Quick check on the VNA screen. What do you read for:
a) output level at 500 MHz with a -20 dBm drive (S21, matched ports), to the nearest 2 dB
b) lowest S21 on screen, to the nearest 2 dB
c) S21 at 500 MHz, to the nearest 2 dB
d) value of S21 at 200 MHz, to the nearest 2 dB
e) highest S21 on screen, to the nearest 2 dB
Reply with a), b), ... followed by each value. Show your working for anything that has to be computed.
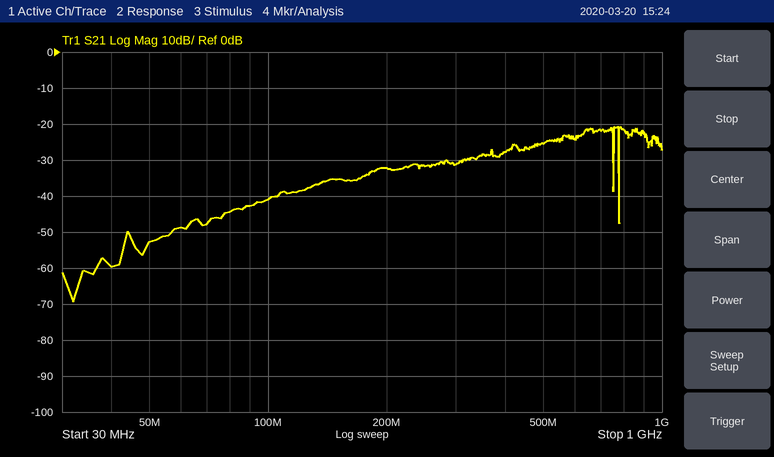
a) -20 dBm + (-26 dB) = -46 dBm
b) -70 dB
c) -26 dB
d) -32 dB
e) -20 dB
